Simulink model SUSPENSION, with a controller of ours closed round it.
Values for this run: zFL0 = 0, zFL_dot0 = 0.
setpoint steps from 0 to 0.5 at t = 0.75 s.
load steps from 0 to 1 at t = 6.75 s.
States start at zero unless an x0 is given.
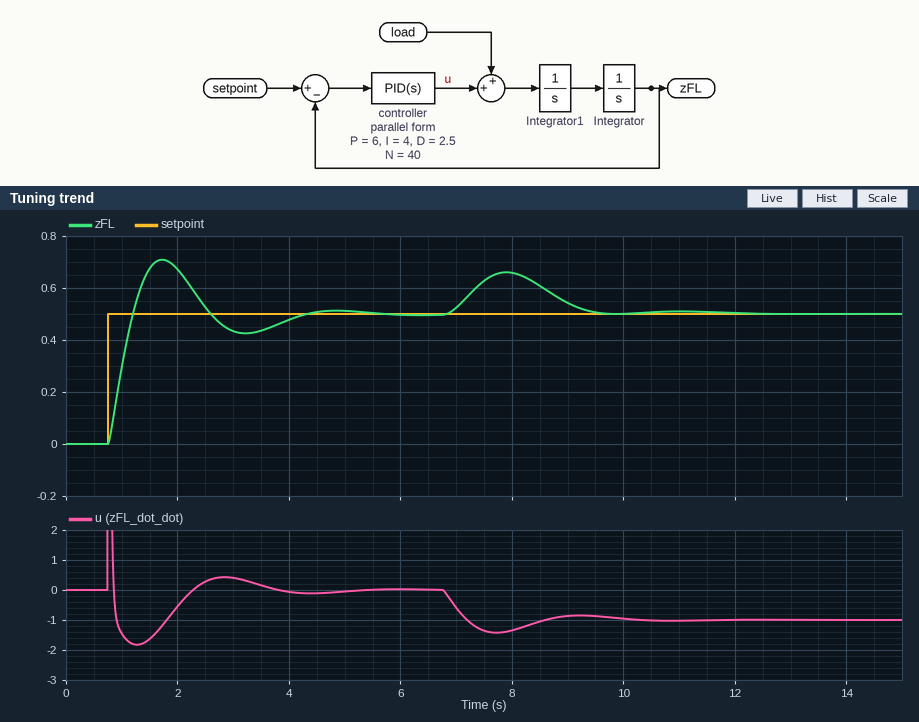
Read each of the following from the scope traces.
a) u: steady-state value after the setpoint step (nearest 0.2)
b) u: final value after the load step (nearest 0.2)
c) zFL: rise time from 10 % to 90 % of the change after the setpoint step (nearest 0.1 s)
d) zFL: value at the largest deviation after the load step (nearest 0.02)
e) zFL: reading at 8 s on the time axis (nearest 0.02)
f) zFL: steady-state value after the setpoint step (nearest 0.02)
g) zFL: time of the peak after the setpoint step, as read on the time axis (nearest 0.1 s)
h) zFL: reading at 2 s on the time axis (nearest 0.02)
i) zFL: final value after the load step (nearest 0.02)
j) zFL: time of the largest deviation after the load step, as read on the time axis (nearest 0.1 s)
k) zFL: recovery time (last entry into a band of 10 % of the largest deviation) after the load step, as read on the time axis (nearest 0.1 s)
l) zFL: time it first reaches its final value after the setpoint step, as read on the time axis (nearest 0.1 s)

0.0
-1.0
0.3 s
0.66
0.66
0.50
1.7 s
0.68
0.50
7.9 s
9.3 s
1.2 s
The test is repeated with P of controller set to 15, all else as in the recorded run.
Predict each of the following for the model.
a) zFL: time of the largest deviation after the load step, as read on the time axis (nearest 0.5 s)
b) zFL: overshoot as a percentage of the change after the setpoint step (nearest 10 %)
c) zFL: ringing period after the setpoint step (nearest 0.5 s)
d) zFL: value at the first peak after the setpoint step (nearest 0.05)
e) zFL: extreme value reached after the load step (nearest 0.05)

7.5 s
50 %
1.5 s
0.75
0.60
